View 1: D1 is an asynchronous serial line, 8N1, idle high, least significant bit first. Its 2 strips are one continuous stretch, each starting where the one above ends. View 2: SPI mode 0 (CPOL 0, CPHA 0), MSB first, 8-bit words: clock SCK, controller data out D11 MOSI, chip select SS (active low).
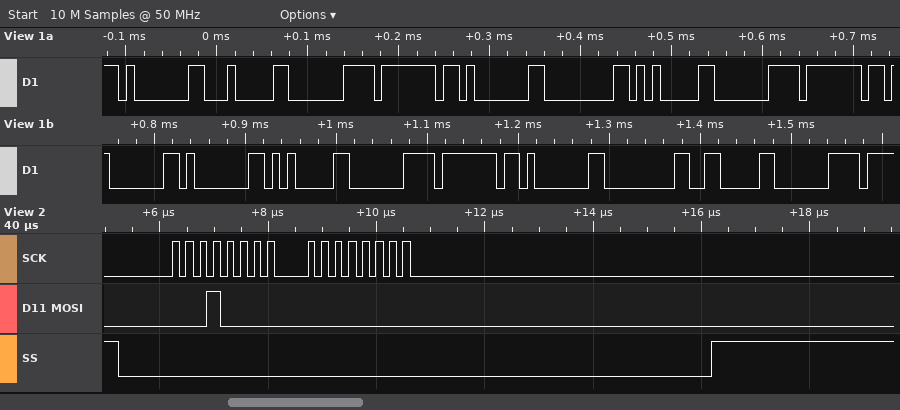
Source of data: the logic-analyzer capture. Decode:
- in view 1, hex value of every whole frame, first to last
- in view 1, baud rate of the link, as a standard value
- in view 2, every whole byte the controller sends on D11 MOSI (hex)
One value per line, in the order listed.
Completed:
0x01 0x04 0xC0 0x7F 0x01 0x00 0x05 0xC0 0x7F 0x01 0x01 0x05 0xC0 0x7F 0x01 0x00 0x06 0xC0
115200 baud
0x10 0x00
